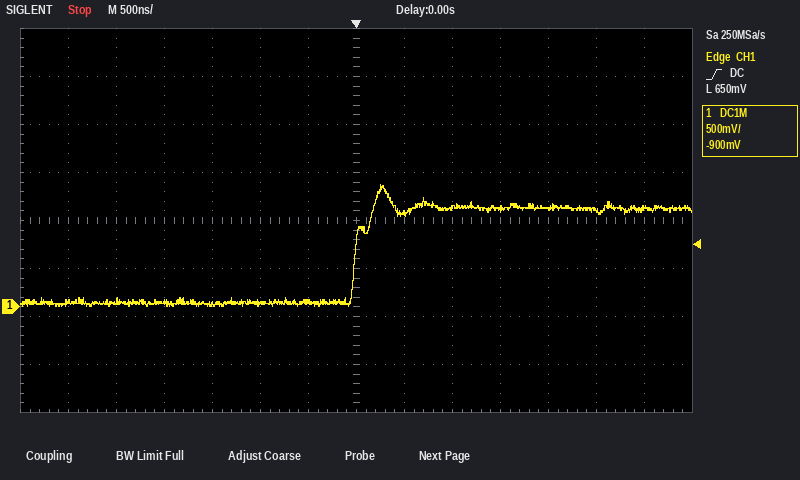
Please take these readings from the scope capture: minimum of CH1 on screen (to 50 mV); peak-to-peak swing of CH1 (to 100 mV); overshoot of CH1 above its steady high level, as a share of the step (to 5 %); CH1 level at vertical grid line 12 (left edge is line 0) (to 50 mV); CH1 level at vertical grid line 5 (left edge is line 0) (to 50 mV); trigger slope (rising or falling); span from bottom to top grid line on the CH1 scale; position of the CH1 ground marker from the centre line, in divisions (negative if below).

0 mV
1.30 V
25 %
1.00 V
50 mV
rising
4 V
-1.8 div
